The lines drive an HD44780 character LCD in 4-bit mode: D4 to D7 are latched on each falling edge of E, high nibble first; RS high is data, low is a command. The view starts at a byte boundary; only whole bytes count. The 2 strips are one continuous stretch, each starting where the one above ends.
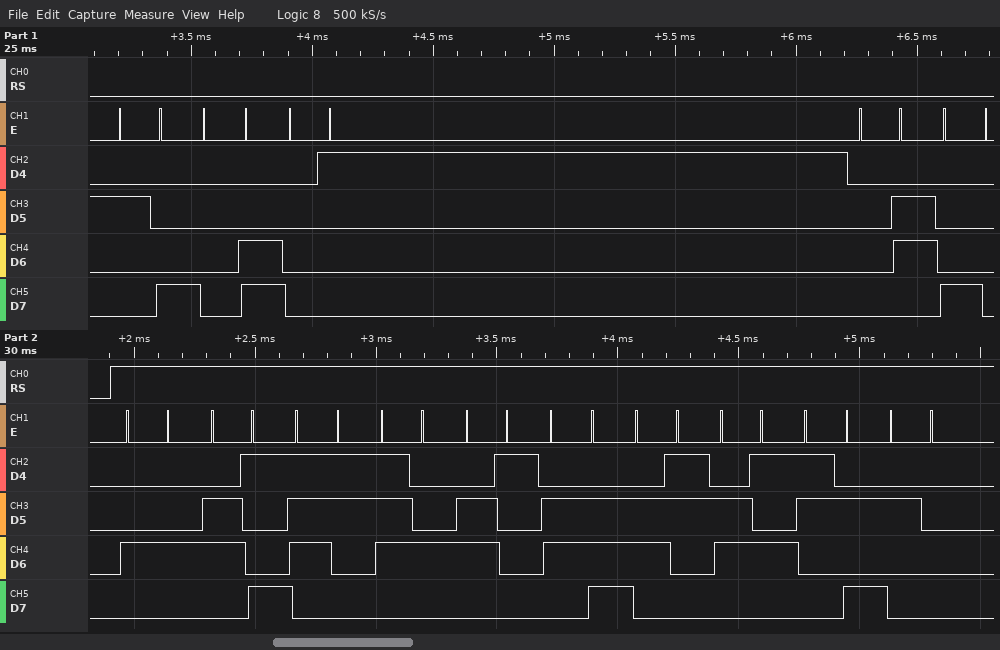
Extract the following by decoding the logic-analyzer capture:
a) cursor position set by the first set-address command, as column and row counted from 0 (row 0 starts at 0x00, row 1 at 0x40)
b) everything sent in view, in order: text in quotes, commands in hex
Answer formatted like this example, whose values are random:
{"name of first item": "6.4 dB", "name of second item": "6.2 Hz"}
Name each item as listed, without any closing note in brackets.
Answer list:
{"cursor position set by the first set-address command, as column and row counted from 0": "column 0, row 0", "everything sent in view, in order: text in quotes, commands in hex": "0x28 0x0C 0x01 0x06 0x80 \"Distance: \""}
